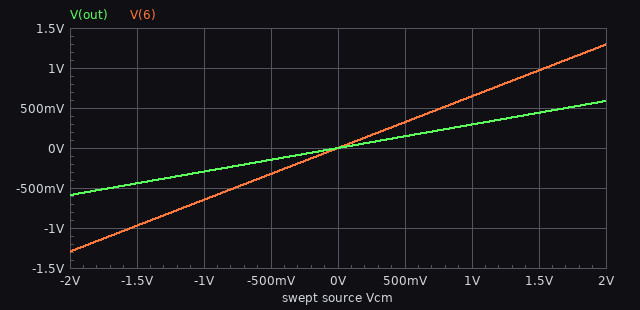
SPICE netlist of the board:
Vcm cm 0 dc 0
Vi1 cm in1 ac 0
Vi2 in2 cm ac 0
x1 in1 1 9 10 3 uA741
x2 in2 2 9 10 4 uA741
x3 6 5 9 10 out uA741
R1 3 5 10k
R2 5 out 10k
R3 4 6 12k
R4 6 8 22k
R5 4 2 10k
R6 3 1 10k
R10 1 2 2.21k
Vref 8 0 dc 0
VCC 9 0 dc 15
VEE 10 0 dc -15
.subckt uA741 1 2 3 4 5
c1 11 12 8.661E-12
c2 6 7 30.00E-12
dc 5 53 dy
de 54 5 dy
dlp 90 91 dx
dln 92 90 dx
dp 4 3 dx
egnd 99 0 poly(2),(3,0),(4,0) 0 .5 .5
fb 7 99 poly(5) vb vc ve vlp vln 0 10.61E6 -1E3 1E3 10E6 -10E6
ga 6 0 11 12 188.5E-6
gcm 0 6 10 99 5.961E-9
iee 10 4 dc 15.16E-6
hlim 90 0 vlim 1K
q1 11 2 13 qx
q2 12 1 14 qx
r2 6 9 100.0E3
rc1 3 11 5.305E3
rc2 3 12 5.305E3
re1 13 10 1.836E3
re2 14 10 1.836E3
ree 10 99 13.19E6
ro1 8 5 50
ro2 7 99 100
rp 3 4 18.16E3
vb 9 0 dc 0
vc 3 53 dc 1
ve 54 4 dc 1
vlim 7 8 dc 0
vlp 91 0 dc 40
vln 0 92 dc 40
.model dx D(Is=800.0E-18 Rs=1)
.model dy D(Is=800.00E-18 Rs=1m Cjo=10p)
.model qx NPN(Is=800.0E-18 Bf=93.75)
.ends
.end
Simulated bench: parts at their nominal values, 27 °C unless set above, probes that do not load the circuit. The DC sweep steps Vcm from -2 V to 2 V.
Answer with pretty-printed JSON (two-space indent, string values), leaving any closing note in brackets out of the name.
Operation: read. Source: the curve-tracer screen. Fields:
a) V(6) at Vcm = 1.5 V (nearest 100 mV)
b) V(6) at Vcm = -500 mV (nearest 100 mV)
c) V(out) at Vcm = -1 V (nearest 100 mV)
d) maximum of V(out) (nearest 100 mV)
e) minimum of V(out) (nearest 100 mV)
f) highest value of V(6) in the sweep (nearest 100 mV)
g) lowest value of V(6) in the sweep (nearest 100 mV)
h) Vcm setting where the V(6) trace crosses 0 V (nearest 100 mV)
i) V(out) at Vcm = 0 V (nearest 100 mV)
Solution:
{
  "V(6) at Vcm = 1.5 V": "1.0 V",
  "V(6) at Vcm = -500 mV": "-300 mV",
  "V(out) at Vcm = -1 V": "-300 mV",
  "maximum of V(out)": "600 mV",
  "minimum of V(out)": "-600 mV",
  "highest value of V(6) in the sweep": "1.3 V",
  "lowest value of V(6) in the sweep": "-1.3 V",
  "Vcm setting where the V(6) trace crosses 0 V": "0 V",
  "V(out) at Vcm = 0 V": "0 V"
}
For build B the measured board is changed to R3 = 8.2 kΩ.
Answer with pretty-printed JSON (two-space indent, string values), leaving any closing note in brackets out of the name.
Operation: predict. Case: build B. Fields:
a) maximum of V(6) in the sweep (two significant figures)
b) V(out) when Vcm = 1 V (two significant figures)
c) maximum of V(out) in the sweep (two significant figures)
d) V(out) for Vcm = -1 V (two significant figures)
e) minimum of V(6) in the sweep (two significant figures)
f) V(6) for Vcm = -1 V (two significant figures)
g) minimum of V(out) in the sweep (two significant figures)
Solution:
{
  "maximum of V(6) in the sweep": "1.5 V",
  "V(out) when Vcm = 1 V": "460 mV",
  "maximum of V(out) in the sweep": "910 mV",
  "V(out) for Vcm = -1 V": "-460 mV",
  "minimum of V(6) in the sweep": "-1.5 V",
  "V(6) for Vcm = -1 V": "-730 mV",
  "minimum of V(out) in the sweep": "-910 mV"
}
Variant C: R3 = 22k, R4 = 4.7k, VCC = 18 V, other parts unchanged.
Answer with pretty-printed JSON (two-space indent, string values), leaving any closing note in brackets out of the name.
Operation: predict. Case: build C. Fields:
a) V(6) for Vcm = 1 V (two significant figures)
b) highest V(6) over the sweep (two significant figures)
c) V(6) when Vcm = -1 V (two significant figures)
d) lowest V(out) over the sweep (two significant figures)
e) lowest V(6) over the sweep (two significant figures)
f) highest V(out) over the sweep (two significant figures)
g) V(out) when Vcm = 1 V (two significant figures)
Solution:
{
  "V(6) for Vcm = 1 V": "180 mV",
  "highest V(6) over the sweep": "350 mV",
  "V(6) when Vcm = -1 V": "-180 mV",
  "lowest V(out) over the sweep": "-1.3 V",
  "lowest V(6) over the sweep": "-350 mV",
  "highest V(out) over the sweep": "1.3 V",
  "V(out) when Vcm = 1 V": "-650 mV"
}
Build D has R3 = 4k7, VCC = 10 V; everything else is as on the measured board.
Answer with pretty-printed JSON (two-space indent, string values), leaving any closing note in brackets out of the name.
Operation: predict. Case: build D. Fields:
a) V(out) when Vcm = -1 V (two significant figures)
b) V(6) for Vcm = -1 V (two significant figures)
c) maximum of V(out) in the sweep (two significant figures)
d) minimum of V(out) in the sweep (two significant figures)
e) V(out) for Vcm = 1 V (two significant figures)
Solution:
{
  "V(out) when Vcm = -1 V": "-650 mV",
  "V(6) for Vcm = -1 V": "-820 mV",
  "maximum of V(out) in the sweep": "1.3 V",
  "minimum of V(out) in the sweep": "-1.3 V",
  "V(out) for Vcm = 1 V": "650 mV"
}
